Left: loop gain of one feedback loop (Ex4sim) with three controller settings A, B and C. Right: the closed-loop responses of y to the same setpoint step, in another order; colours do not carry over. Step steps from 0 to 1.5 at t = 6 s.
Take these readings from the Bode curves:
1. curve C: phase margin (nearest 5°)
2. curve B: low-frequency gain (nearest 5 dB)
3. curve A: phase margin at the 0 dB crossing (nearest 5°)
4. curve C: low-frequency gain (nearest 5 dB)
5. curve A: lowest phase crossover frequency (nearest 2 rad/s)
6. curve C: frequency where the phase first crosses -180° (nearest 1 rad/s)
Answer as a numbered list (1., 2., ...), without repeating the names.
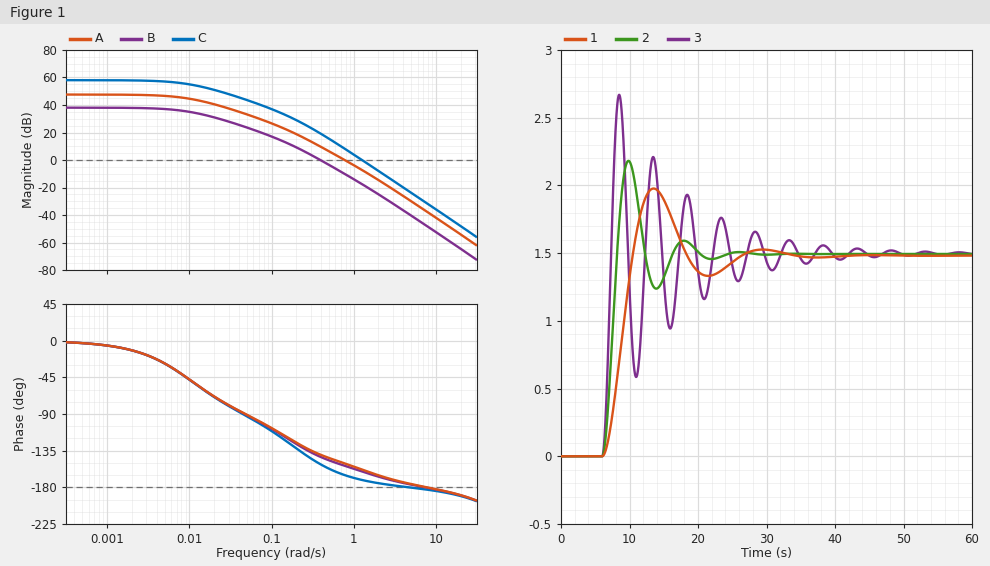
1. 10°
2. 40 dB
3. 30°
4. 60 dB
5. 8 rad/s
6. 5 rad/s
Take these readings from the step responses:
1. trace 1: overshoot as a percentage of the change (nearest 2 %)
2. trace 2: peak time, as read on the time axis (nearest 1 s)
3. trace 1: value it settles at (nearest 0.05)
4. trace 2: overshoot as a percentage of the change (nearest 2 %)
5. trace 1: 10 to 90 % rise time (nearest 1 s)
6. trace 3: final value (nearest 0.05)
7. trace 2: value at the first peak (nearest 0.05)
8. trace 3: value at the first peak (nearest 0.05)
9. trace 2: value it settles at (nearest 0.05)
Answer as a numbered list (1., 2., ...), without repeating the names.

1. 34 %
2. 10 s
3. 1.50
4. 46 %
5. 3 s
6. 1.50
7. 2.20
8. 2.65
9. 1.50
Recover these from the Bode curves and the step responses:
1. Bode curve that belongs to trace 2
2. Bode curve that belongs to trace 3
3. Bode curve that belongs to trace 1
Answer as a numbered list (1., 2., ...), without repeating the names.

1. A
2. C
3. B
